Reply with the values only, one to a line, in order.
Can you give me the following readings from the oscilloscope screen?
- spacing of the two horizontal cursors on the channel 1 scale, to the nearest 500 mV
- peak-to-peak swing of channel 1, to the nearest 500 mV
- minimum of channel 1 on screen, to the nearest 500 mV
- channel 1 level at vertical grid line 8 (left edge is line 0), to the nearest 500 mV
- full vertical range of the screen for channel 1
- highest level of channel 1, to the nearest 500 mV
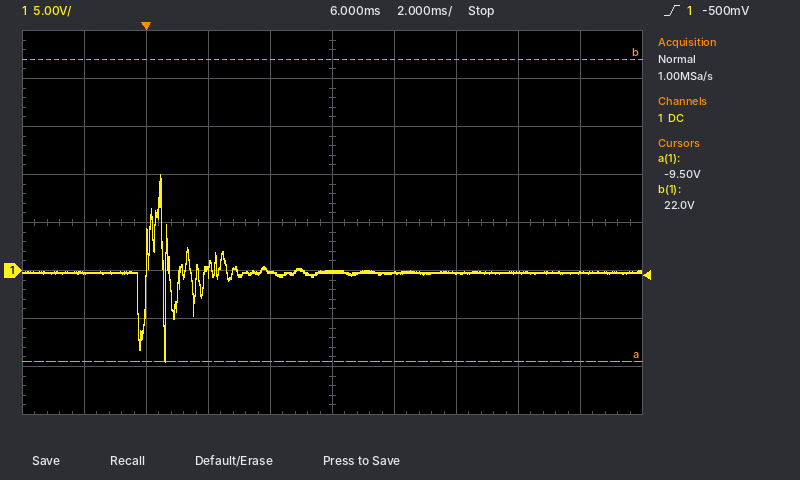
31.5 V
19.5 V
-9.5 V
0.0 V
40 V
10.0 V
